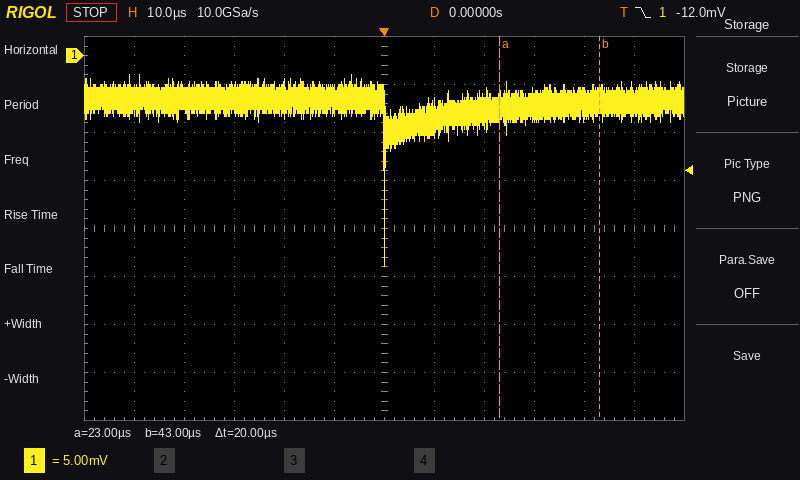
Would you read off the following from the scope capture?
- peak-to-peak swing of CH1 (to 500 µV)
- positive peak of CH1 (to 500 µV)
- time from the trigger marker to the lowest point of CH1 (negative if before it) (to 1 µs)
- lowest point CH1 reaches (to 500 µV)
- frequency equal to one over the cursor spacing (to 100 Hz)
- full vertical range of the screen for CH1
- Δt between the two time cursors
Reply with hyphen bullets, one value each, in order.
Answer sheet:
- 20.0 mV
- -2.0 mV
- 0 µs
- -22.0 mV
- 50.0 kHz
- 40 mV
- 20 µs
